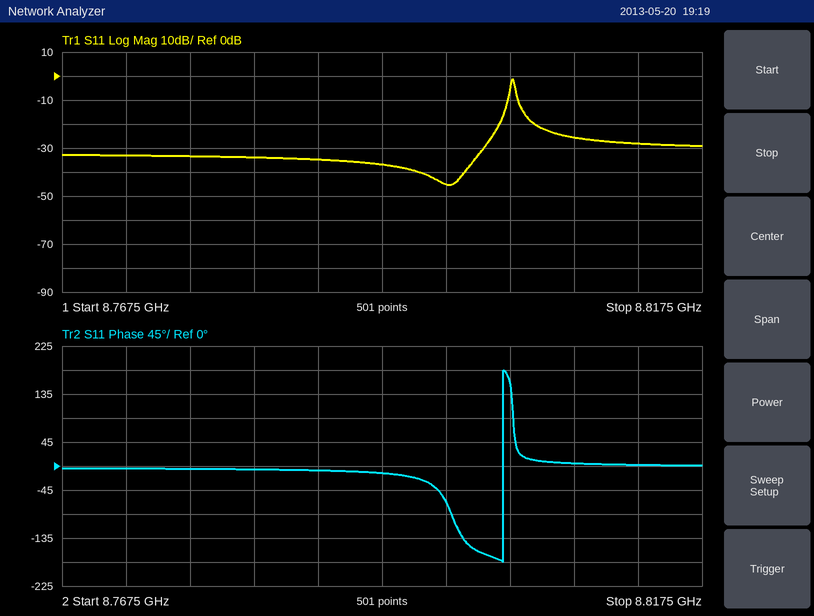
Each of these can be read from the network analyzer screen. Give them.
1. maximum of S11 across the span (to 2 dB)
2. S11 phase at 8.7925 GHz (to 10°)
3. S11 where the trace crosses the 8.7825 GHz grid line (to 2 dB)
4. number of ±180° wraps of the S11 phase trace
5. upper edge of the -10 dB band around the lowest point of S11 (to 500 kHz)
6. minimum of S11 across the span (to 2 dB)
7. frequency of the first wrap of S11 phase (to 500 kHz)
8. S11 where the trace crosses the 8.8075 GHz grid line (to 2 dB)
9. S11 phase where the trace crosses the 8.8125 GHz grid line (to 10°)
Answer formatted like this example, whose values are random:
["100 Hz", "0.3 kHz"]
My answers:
["-2 dB", "-10°", "-34 dB", "1", "8.8025 GHz", "-46 dB", "8.8020 GHz", "-26 dB", "0°"]
